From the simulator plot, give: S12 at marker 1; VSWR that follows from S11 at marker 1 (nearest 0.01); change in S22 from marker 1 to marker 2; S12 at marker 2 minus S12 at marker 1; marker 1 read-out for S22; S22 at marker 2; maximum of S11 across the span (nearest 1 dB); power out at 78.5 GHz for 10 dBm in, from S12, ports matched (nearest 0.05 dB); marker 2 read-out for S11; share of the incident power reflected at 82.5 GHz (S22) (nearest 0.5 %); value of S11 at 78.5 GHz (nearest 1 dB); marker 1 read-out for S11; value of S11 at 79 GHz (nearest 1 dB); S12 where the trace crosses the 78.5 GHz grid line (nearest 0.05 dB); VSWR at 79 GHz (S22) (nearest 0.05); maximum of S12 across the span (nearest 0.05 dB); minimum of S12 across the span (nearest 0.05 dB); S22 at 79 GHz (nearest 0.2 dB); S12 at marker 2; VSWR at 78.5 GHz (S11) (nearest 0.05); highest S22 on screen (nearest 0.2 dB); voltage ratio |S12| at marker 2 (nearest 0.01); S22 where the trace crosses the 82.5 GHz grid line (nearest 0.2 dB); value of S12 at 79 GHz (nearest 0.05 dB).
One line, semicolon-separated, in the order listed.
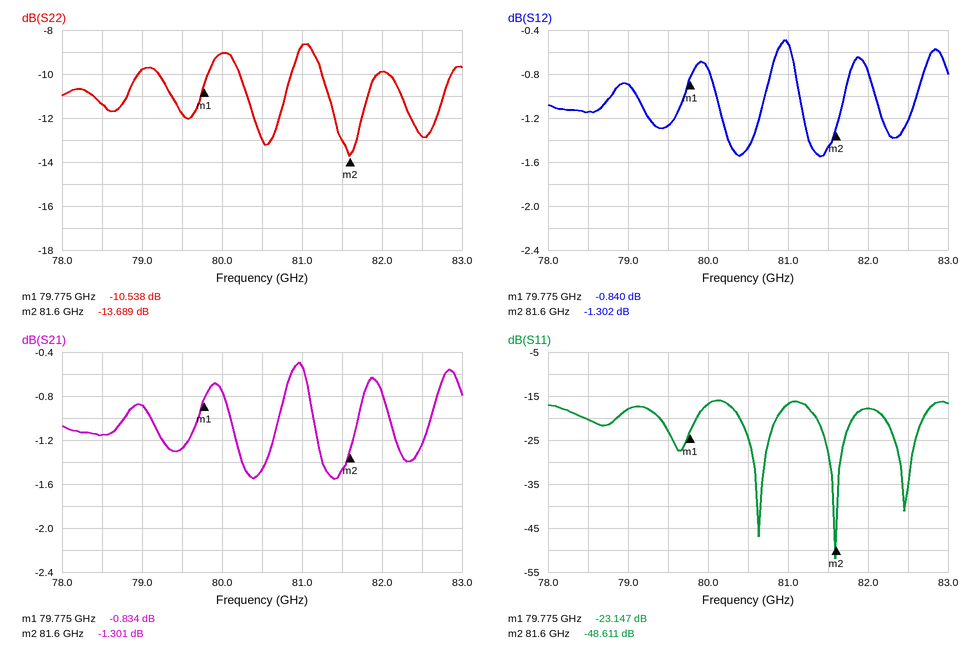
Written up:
-0.840 dB; 1.15; -3.151 dB; -0.462 dB; -10.538 dB; -13.689 dB; -16 dB; 8.85 dBm; -48.611 dB; 5.0 %; -20 dB; -23.147 dB; -18 dB; -1.15 dB; 1.95; -0.50 dB; -1.55 dB; -9.8 dB; -1.302 dB; 1.20; -8.6 dB; 0.86; -12.8 dB; -0.90 dB
